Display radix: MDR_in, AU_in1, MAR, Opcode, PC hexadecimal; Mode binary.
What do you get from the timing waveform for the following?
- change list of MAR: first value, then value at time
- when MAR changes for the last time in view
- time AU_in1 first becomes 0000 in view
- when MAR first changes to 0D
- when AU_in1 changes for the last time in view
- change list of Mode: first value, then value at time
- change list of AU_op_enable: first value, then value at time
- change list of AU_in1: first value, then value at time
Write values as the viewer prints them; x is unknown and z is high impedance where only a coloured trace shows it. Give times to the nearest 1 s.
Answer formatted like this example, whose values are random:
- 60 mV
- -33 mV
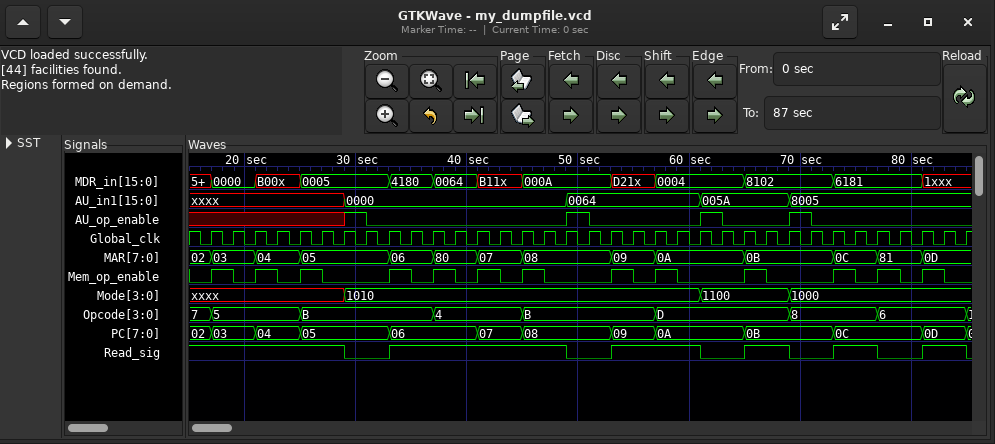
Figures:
- 02, 03 at 17 s, 04 at 21 s, 05 at 25 s, 06 at 33 s, 80 at 37 s, 07 at 41 s, 08 at 45 s, 09 at 53 s, 0A at 57 s, 0B at 65 s, 0C at 73 s, 81 at 77 s, 0D at 81 s
- 81 s
- 29 s
- 81 s
- 69 s
- xxxx, 1010 at 29 s, 1100 at 61 s, 1000 at 69 s
- x, 1 at 29 s, 0 at 31 s, 1 at 49 s, 0 at 51 s, 1 at 61 s, 0 at 63 s, 1 at 69 s, 0 at 71 s
- xxxx, 0000 at 29 s, 0064 at 49 s, 005A at 61 s, 8005 at 69 s
